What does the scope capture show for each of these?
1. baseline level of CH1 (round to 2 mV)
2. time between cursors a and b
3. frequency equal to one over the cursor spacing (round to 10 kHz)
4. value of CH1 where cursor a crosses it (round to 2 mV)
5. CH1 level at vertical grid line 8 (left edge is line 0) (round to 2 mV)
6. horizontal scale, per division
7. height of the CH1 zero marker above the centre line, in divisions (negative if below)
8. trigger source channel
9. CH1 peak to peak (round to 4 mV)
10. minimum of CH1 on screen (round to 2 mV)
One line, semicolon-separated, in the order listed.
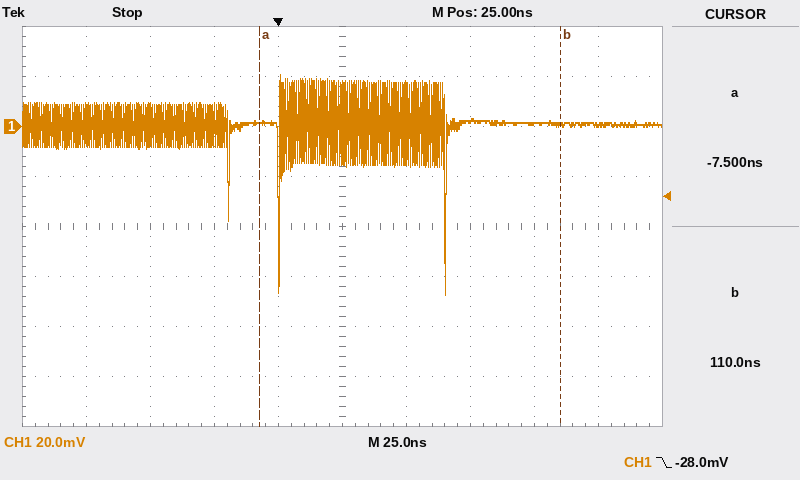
2 mV; 117.5 ns; 8.51 MHz; 2 mV; 2 mV; 25 ns; +2.0 div; CH1; 88 mV; -68 mV
